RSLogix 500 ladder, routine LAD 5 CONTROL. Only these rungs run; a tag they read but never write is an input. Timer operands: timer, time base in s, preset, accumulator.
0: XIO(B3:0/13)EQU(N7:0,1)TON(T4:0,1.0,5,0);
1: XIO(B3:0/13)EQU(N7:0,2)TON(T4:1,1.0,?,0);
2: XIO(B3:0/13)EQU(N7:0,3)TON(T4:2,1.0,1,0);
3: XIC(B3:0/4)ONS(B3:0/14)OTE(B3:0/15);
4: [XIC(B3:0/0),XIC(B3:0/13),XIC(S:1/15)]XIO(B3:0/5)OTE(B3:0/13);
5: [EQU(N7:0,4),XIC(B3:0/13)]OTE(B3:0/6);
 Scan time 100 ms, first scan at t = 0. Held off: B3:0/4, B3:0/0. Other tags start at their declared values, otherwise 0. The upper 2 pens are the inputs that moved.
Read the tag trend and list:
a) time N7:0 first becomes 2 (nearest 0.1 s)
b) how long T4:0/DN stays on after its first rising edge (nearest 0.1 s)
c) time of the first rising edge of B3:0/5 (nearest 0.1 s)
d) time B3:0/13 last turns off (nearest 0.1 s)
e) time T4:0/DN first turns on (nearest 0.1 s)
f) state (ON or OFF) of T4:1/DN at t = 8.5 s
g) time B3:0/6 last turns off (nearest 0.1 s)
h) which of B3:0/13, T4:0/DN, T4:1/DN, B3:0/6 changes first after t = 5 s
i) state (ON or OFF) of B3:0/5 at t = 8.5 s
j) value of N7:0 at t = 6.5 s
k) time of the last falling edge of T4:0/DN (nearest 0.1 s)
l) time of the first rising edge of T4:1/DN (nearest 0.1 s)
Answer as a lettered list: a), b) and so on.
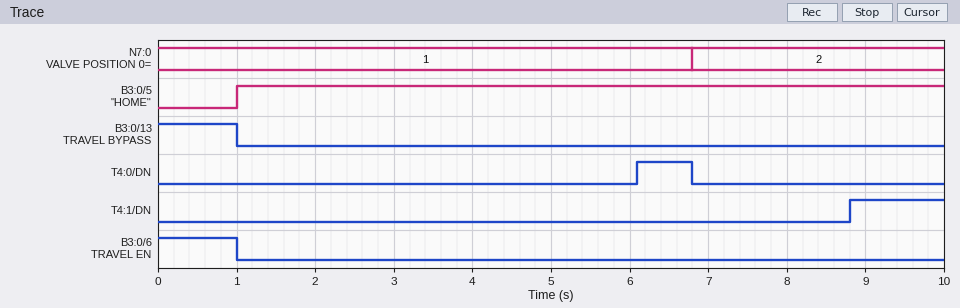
a) 6.8 s
b) 0.7 s
c) 1.0 s
d) 1.0 s
e) 6.1 s
f) OFF
g) 1.0 s
h) T4:0/DN
i) ON
j) 1
k) 6.8 s
l) 8.8 s
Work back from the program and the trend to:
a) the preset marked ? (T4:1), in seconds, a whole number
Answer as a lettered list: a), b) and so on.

a) 2 s
